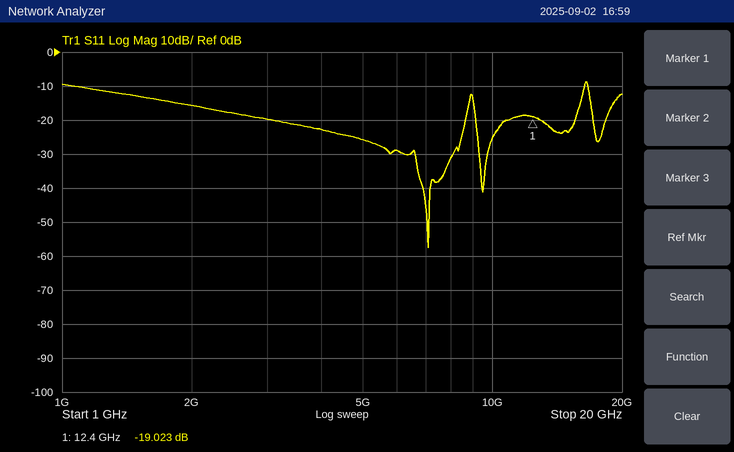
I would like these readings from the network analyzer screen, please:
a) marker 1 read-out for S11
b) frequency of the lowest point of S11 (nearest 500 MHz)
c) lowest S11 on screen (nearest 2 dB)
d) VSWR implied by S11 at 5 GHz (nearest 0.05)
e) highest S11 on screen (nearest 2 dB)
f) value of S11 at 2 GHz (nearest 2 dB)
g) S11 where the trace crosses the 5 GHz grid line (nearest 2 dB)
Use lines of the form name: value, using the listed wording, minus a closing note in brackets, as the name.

marker 1 read-out for S11: -19.023 dB
frequency of the lowest point of S11: 7.0 GHz
lowest S11 on screen: -58 dB
VSWR implied by S11 at 5 GHz: 1.10
highest S11 on screen: -8 dB
value of S11 at 2 GHz: -16 dB
S11 where the trace crosses the 5 GHz grid line: -26 dB
